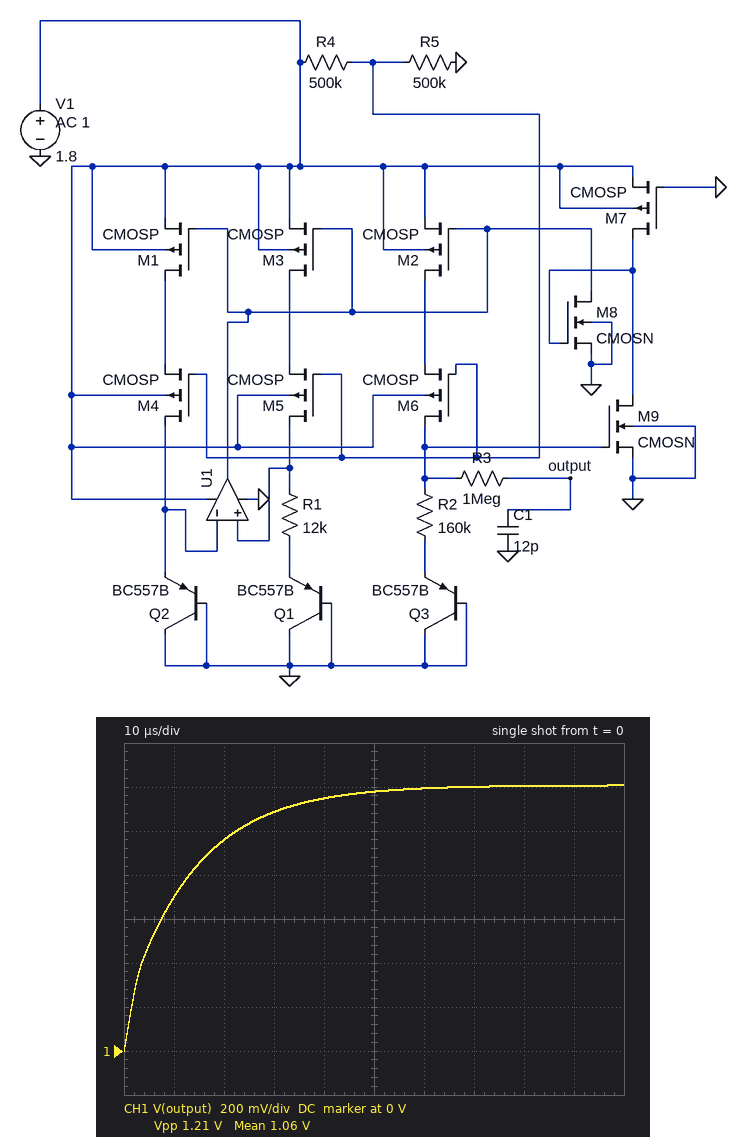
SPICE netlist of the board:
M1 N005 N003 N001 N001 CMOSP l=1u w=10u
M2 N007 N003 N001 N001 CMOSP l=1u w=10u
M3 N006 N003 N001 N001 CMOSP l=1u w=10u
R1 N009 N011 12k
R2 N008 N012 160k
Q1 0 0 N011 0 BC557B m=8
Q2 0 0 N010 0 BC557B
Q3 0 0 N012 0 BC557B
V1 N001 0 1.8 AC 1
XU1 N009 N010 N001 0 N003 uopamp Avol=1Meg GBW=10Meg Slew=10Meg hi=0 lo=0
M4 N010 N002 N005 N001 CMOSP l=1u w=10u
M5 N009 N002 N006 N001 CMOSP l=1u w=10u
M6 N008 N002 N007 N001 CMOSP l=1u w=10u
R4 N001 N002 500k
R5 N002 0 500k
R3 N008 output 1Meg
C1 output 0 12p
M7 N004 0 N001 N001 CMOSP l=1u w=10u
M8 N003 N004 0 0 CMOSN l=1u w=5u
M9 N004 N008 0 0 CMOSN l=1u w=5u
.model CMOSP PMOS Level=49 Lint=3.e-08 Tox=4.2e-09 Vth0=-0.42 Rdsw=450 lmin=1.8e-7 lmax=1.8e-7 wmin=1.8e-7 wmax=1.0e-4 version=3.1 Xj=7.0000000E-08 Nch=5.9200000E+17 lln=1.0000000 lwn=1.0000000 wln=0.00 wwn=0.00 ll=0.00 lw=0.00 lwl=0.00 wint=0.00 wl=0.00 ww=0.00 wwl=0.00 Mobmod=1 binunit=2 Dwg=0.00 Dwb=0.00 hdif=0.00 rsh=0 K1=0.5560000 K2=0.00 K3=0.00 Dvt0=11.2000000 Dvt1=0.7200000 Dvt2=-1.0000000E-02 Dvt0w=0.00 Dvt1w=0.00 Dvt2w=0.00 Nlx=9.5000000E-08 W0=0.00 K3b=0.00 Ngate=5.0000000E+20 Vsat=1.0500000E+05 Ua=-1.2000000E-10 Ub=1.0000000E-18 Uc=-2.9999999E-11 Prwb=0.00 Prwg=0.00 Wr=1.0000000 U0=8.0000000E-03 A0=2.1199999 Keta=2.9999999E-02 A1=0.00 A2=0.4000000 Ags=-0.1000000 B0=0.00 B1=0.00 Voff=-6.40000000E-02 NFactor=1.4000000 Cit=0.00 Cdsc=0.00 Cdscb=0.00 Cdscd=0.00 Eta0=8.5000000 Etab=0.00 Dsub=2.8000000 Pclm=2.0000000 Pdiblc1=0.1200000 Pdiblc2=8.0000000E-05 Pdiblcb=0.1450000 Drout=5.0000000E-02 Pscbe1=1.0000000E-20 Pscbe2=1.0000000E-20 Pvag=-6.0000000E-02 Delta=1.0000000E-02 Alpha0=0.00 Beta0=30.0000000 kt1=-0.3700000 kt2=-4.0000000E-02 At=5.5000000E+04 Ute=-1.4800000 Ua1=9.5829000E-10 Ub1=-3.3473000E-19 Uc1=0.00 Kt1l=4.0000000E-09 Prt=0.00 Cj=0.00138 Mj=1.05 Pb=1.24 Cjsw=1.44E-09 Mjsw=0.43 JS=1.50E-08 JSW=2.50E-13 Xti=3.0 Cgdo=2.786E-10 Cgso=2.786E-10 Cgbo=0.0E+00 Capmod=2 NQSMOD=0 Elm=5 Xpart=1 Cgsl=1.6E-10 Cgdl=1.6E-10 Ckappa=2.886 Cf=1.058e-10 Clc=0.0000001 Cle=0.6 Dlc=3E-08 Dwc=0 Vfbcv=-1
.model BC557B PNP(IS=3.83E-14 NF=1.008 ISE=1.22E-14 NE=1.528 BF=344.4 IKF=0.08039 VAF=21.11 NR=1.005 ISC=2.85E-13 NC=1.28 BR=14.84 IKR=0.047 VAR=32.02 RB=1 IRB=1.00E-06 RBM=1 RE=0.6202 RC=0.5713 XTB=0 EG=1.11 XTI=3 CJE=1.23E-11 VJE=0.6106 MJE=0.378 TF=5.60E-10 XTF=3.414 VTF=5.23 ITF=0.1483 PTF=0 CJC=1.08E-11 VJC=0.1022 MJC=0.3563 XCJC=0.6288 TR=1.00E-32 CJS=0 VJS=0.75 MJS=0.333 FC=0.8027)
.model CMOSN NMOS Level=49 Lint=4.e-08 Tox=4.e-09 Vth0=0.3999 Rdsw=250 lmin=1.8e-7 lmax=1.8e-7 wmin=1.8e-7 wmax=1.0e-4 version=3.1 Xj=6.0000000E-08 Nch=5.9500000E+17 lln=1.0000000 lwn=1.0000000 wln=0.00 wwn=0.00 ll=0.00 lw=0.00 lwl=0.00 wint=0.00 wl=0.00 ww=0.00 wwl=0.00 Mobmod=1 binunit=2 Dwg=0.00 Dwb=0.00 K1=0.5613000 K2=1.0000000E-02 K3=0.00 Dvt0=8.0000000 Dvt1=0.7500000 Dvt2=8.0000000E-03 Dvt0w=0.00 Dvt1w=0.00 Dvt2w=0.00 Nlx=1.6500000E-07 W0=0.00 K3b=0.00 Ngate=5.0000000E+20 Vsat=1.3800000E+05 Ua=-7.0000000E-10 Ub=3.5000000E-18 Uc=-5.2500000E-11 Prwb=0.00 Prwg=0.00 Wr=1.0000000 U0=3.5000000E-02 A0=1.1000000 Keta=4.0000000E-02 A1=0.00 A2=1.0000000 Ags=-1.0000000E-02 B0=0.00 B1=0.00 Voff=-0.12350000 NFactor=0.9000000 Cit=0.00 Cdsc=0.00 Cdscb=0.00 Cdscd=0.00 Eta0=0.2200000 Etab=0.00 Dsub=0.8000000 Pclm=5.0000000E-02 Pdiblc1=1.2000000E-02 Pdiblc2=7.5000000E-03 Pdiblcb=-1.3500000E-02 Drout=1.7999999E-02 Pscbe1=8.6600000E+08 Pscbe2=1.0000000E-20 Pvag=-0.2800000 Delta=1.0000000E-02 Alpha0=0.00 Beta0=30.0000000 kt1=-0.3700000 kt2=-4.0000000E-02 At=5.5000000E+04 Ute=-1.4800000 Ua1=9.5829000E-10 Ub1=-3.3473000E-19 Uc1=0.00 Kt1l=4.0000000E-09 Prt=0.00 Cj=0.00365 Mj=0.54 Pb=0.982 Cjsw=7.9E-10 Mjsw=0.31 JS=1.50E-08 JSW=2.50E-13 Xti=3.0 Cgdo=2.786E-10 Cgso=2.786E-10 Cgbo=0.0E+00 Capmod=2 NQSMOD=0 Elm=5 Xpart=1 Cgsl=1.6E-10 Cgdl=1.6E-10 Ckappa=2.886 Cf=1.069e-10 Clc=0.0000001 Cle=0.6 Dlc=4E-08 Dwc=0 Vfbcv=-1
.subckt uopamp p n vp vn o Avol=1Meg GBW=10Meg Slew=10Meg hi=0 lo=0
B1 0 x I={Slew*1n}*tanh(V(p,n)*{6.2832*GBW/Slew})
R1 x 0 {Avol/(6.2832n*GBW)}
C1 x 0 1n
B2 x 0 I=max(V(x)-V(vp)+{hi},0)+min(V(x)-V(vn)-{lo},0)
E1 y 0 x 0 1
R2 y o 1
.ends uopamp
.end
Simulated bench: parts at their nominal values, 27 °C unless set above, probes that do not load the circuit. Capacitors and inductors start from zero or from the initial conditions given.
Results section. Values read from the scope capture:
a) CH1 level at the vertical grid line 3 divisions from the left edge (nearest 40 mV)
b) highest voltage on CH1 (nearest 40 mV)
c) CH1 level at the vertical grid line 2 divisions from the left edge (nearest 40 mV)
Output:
1.08 V
1.20 V
960 mV
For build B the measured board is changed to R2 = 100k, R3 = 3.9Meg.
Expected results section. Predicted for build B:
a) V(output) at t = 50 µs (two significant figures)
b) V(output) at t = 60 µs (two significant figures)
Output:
620 mV
680 mV
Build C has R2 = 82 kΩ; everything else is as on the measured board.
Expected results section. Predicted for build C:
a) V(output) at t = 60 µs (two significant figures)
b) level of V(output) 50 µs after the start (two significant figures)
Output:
850 mV
840 mV
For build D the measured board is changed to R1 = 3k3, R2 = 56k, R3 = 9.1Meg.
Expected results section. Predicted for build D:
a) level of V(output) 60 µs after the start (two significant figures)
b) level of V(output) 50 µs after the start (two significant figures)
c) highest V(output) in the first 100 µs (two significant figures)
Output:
600 mV
520 mV
850 mV
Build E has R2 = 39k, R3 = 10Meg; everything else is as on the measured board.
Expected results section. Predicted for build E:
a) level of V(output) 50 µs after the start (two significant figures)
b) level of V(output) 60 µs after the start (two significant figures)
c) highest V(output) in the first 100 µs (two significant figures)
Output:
230 mV
270 mV
380 mV
